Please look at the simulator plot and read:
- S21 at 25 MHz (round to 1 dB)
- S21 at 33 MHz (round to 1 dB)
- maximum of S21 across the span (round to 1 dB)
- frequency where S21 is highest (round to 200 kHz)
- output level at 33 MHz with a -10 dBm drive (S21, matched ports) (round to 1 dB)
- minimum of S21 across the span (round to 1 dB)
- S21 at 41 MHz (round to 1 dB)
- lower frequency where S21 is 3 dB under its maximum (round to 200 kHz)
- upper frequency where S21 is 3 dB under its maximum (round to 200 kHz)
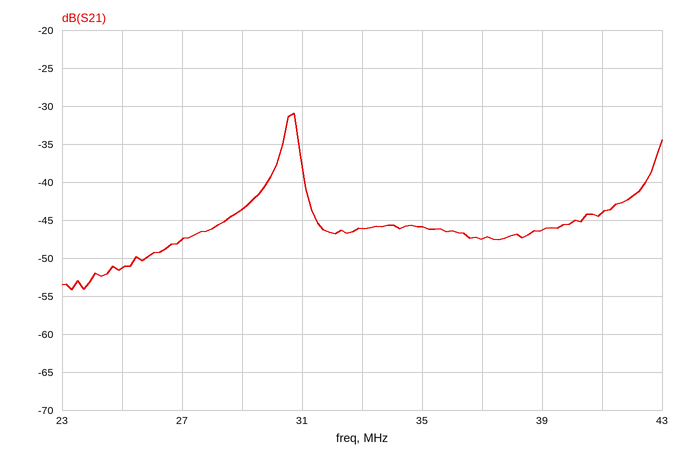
-51 dB
-46 dB
-31 dB
30.8 MHz
-56 dBm
-54 dB
-44 dB
30.4 MHz
30.8 MHz
